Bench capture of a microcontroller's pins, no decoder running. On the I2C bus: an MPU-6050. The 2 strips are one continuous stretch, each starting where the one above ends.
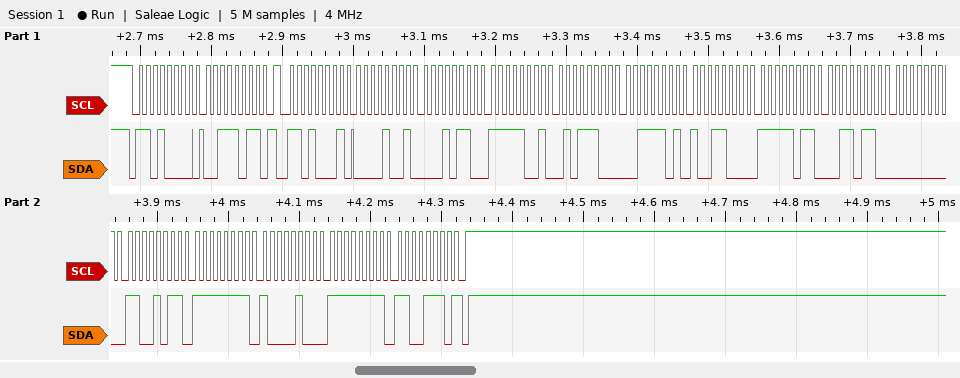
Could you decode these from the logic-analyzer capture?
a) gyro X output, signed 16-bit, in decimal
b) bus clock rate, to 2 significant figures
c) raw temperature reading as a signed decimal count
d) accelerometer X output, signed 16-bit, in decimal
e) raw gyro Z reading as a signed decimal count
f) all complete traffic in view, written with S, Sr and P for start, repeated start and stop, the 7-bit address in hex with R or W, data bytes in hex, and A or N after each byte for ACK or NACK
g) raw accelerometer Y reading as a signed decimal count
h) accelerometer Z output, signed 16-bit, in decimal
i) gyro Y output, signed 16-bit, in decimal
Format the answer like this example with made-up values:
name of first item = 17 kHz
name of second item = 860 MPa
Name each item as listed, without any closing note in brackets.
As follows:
gyro X output, signed 16-bit, in decimal = 203
bus clock rate, to 2 significant figures = 100 kHz
raw temperature reading as a signed decimal count = -1226
accelerometer X output, signed 16-bit, in decimal = 2326
raw gyro Z reading as a signed decimal count = -50
all complete traffic in view, written with S, Sr and P for start, repeated start and stop, the 7-bit address in hex with R or W, data bytes in hex, and A or N after each byte for ACK or NACK = S 68W A 3B A Sr 68R A 09 A 16 A F9 A 5C A 3D A 98 A FB A 36 A 00 A CB A FF A 84 A FF A CE N P
raw accelerometer Y reading as a signed decimal count = -1700
accelerometer Z output, signed 16-bit, in decimal = 15768
gyro Y output, signed 16-bit, in decimal = -124
